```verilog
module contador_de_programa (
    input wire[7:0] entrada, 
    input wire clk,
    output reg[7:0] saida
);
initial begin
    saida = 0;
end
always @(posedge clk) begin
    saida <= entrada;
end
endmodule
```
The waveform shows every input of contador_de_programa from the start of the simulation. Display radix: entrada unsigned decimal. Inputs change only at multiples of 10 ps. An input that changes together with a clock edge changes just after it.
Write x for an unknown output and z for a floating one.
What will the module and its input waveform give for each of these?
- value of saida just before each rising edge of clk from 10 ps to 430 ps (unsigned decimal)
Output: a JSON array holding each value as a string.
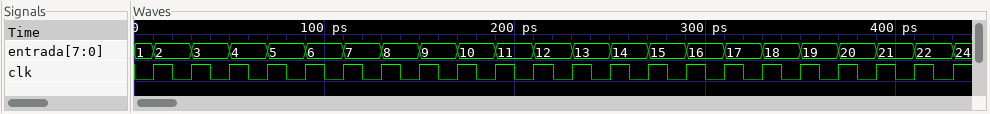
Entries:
["0, 1, 2, 3, 4, 5, 6, 7, 8, 9, 10, 11, 12, 13, 14, 15, 16, 17, 18, 19, 20, 21"]
